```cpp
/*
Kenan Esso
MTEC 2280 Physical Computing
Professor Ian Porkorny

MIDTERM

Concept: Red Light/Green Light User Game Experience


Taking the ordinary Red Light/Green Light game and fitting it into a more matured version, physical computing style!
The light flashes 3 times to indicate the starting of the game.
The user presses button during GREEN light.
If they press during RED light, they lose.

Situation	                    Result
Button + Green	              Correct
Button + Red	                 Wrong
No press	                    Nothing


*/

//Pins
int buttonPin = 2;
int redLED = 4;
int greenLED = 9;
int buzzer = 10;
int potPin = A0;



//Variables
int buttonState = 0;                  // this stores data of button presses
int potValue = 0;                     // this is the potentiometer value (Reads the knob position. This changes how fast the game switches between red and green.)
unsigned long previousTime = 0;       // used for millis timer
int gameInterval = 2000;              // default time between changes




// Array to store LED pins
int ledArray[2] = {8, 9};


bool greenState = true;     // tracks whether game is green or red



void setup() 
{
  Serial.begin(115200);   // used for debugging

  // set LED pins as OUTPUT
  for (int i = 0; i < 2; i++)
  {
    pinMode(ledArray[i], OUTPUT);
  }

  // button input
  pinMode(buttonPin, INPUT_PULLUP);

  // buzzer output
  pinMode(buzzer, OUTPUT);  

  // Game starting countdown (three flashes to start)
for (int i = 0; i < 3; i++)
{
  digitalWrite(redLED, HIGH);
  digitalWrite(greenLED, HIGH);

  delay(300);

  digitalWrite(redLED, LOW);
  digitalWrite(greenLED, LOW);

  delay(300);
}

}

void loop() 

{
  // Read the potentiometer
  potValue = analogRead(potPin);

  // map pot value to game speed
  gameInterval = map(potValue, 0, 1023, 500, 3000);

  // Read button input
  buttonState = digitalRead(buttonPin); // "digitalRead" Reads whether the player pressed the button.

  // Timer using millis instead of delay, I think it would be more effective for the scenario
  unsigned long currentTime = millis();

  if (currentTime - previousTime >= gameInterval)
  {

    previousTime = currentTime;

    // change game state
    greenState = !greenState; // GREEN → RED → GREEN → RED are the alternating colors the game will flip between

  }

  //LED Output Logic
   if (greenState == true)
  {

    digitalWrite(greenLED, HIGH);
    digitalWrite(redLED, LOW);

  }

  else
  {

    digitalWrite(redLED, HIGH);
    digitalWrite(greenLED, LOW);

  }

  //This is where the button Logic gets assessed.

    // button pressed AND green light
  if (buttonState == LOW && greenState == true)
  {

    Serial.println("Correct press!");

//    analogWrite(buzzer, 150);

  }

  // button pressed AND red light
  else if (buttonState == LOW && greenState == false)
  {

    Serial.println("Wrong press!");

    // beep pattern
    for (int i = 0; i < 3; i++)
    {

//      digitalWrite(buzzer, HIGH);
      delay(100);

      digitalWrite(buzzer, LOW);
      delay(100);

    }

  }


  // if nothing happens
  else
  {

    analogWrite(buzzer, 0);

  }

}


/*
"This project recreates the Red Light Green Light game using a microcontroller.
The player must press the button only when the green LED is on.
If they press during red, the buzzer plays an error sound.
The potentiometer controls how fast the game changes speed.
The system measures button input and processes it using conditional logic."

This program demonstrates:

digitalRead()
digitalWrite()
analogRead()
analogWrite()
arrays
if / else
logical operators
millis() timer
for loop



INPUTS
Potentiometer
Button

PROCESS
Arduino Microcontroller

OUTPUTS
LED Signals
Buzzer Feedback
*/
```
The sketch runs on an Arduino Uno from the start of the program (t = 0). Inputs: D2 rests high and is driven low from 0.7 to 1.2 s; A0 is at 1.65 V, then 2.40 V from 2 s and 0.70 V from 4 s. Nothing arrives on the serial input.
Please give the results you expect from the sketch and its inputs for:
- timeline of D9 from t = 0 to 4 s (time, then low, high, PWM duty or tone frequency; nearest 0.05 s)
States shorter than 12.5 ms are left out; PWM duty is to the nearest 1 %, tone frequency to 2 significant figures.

0 s high; 0.3 s low; 0.6 s high; 0.9 s low; 1.2 s high; 1.5 s low; 3.5 s high
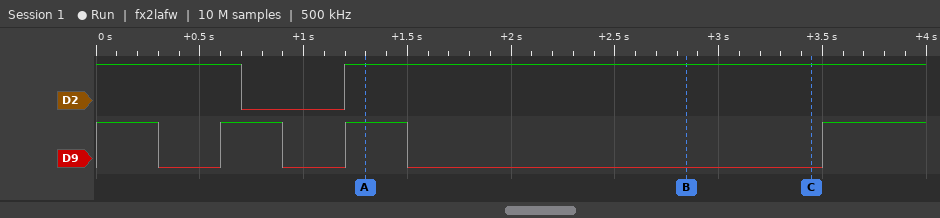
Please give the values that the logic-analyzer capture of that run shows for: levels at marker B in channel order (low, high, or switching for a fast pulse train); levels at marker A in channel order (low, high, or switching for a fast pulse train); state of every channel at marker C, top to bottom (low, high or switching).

D2 high, D9 low
D2 high, D9 high
D2 high, D9 low
